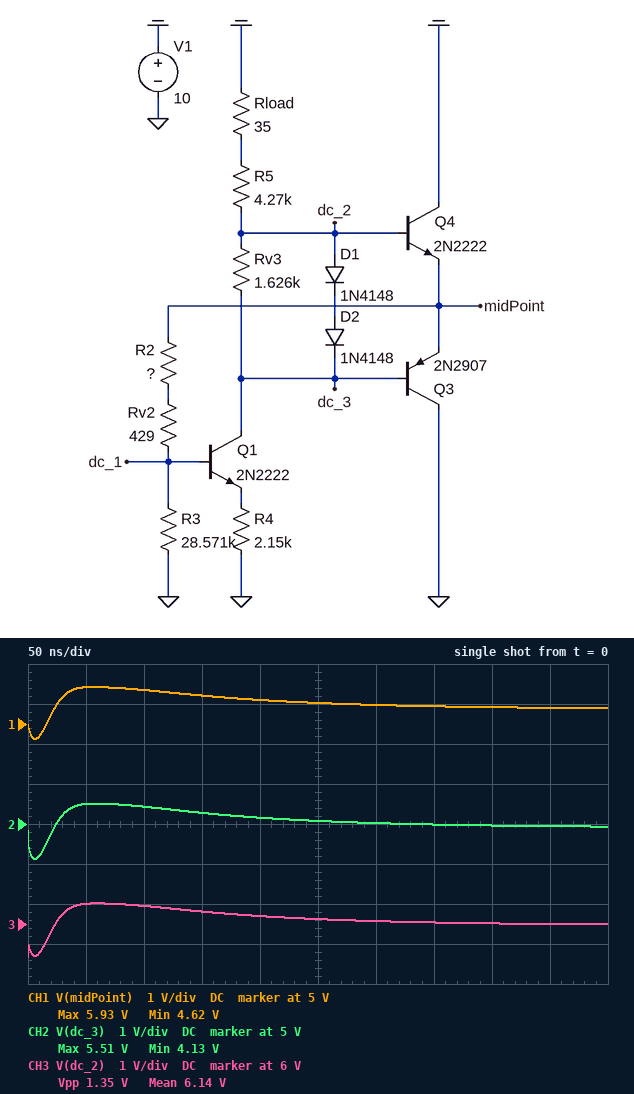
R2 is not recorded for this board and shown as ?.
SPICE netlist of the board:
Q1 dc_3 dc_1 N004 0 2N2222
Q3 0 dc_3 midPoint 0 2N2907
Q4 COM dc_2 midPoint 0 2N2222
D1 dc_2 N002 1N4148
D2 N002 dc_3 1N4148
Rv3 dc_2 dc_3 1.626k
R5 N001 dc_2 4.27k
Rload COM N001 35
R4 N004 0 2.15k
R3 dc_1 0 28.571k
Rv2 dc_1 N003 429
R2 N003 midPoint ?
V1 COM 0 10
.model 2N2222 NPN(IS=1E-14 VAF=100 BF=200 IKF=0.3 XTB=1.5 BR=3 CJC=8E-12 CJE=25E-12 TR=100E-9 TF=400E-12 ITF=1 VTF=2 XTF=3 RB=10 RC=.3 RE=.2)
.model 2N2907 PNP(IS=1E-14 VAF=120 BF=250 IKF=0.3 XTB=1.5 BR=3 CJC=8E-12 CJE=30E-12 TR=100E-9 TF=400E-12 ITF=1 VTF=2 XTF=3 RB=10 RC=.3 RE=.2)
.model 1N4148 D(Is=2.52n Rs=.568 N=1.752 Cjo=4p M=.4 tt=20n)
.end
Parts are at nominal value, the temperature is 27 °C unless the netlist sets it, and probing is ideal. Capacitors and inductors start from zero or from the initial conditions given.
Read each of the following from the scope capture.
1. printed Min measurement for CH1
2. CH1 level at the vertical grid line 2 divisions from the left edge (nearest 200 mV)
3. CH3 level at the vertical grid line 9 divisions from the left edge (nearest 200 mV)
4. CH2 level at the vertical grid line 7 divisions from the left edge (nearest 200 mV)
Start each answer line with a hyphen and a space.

- 4.62 V
- 5.8 V
- 6.0 V
- 5.0 V
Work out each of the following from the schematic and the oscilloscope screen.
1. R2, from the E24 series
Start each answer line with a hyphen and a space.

- 27 kΩ
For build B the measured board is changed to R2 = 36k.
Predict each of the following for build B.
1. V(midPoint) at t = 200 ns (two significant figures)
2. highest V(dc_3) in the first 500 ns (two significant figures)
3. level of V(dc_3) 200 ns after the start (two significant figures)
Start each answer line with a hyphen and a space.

- 5.9 V
- 5.6 V
- 5.5 V
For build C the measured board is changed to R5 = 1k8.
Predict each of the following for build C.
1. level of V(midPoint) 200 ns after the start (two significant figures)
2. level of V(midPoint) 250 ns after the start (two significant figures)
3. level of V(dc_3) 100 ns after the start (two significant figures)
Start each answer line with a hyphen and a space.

- 7.1 V
- 7.0 V
- 6.7 V
